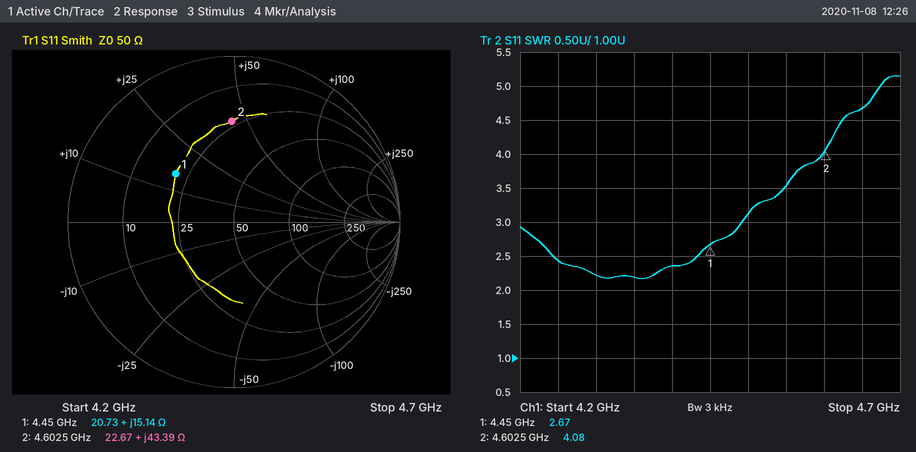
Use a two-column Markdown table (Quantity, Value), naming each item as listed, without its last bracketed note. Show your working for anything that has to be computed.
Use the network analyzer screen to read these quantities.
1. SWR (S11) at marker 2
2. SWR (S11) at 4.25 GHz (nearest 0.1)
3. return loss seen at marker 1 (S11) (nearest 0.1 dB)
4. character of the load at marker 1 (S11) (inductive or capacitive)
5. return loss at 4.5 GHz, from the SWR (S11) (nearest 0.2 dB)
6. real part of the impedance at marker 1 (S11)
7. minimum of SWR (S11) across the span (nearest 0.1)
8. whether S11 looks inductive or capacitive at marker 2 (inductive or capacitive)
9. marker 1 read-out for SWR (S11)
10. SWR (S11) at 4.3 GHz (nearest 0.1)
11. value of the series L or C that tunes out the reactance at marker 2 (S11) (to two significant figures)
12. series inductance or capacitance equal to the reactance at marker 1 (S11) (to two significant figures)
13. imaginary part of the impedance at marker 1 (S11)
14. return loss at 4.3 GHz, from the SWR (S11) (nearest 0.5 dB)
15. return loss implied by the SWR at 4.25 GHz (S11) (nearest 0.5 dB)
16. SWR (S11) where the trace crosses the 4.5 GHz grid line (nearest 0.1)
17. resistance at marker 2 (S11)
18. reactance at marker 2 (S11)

| Quantity | Value |
|---|---|
| SWR (S11) at marker 2 | 4.08 |
| SWR (S11) at 4.25 GHz | 2.4 |
| return loss seen at marker 1 (S11) | 6.8 dB |
| character of the load at marker 1 (S11) | inductive |
| return loss at 4.5 GHz, from the SWR (S11) | −20 log10((3.1 − 1)/(3.1 + 1)) ≈ 5.8 dB |
| real part of the impedance at marker 1 | 20.73 Ω |
| minimum of SWR (S11) across the span | 2.2 |
| whether S11 looks inductive or capacitive at marker 2 | inductive |
| marker 1 read-out for SWR | 2.67 |
| SWR (S11) at 4.3 GHz | 2.2 |
| value of the series L or C that tunes out the reactance at marker 2 (S11) | C = 1/(2π × 4.6025 GHz × 43.39 Ω) ≈ 797 fF, so 800 fF to two significant figures |
| series inductance or capacitance equal to the reactance at marker 1 (S11) | L = 15.14 Ω/(2π × 4.45 GHz) ≈ 541 pH, so 540 pH to two significant figures |
| imaginary part of the impedance at marker 1 | +15.14 Ω |
| return loss at 4.3 GHz, from the SWR (S11) | −20 log10((2.2 − 1)/(2.2 + 1)) ≈ 8.5 dB |
| return loss implied by the SWR at 4.25 GHz (S11) | −20 log10((2.4 − 1)/(2.4 + 1)) ≈ 7.71 dB, so 7.5 dB to the nearest 0.5 dB |
| SWR (S11) where the trace crosses the 4.5 GHz grid line | 3.1 |
| resistance at marker 2 | 22.67 Ω |
| reactance at marker 2 | +43.39 Ω |
